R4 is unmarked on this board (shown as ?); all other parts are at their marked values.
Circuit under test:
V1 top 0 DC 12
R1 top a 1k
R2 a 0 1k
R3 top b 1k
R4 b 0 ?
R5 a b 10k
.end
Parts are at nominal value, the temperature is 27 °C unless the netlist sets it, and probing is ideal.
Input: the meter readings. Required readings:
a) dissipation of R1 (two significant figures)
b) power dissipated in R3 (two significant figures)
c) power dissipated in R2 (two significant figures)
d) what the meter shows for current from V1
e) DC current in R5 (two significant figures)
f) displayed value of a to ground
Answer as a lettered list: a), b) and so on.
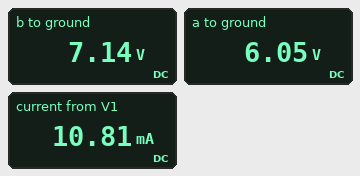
a) 35 mW
b) 24 mW
c) 37 mW
d) 10.81 mA
e) 110 µA
f) 6.05 V
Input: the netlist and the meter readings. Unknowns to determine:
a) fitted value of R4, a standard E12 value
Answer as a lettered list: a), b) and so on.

a) 1.5 kΩ
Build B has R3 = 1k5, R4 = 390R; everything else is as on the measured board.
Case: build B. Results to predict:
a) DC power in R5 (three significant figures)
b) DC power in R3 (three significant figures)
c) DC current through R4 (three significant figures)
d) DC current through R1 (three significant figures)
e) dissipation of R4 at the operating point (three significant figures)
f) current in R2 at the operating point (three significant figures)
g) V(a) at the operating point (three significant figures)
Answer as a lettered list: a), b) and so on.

a) 1.06 mW
b) 59.2 mW
c) 6.61 mA
d) 6.16 mA
e) 17.0 mW
f) 5.84 mA
g) 5.84 V
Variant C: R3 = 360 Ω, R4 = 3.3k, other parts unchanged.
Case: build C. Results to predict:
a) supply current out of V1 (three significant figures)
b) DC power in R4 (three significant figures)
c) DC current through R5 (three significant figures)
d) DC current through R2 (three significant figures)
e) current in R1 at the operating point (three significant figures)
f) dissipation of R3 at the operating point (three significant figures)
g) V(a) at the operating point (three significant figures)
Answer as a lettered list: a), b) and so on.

a) 9.46 mA
b) 34.5 mW
c) 445 µA
d) 6.22 mA
e) 5.78 mA
f) 4.88 mW
g) 6.22 V
